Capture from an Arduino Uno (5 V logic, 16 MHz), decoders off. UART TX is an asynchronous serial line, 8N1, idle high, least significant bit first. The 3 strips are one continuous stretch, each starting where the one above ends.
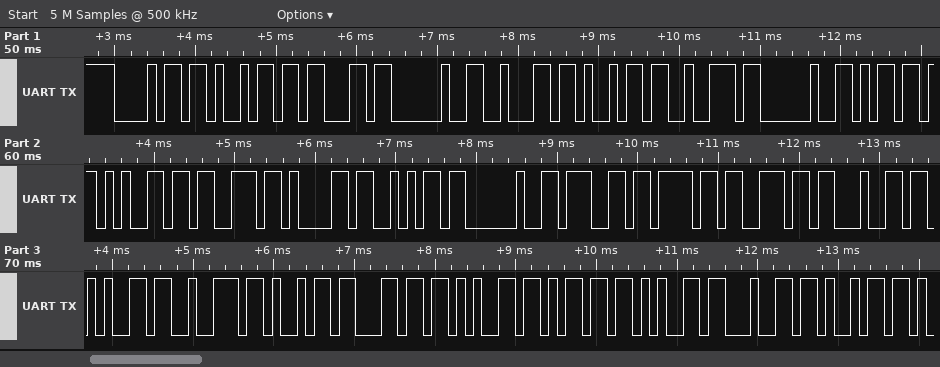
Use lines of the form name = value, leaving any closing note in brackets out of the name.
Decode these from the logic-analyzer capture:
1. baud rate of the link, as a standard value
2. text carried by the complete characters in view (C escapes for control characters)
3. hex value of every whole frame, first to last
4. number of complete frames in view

baud rate of the link, as a standard value = 9600 baud
text carried by the complete characters in view = "hic bir mesaj gonderilemedi"
hex value of every whole frame, first to last = 68 69 63 20 62 69 72 20 6D 65 73 61 6A 20 67 6F 6E 64 65 72 69 6C 65 6D 65 64 69
number of complete frames in view = 27
